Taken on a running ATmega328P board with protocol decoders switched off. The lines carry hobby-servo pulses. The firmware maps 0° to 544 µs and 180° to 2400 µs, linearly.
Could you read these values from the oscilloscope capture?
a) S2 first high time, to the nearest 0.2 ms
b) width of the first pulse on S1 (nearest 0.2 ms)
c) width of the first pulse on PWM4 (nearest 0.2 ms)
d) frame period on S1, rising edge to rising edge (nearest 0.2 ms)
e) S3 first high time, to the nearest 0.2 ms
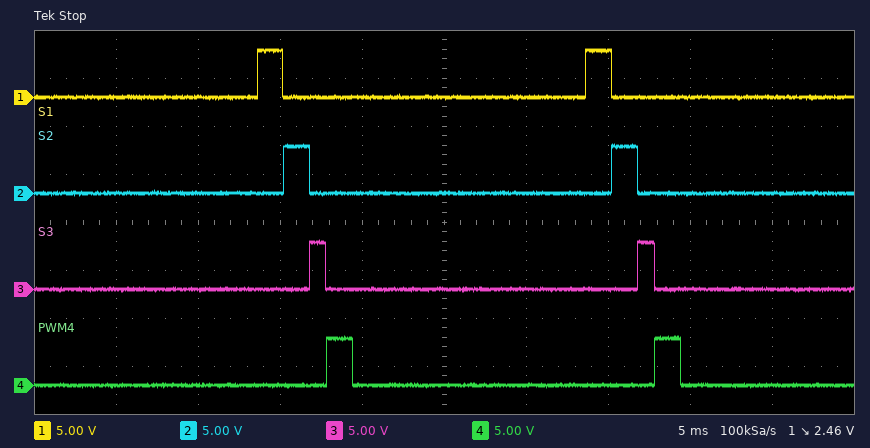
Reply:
1.6 ms
1.6 ms
1.6 ms
20.0 ms
1.0 ms
